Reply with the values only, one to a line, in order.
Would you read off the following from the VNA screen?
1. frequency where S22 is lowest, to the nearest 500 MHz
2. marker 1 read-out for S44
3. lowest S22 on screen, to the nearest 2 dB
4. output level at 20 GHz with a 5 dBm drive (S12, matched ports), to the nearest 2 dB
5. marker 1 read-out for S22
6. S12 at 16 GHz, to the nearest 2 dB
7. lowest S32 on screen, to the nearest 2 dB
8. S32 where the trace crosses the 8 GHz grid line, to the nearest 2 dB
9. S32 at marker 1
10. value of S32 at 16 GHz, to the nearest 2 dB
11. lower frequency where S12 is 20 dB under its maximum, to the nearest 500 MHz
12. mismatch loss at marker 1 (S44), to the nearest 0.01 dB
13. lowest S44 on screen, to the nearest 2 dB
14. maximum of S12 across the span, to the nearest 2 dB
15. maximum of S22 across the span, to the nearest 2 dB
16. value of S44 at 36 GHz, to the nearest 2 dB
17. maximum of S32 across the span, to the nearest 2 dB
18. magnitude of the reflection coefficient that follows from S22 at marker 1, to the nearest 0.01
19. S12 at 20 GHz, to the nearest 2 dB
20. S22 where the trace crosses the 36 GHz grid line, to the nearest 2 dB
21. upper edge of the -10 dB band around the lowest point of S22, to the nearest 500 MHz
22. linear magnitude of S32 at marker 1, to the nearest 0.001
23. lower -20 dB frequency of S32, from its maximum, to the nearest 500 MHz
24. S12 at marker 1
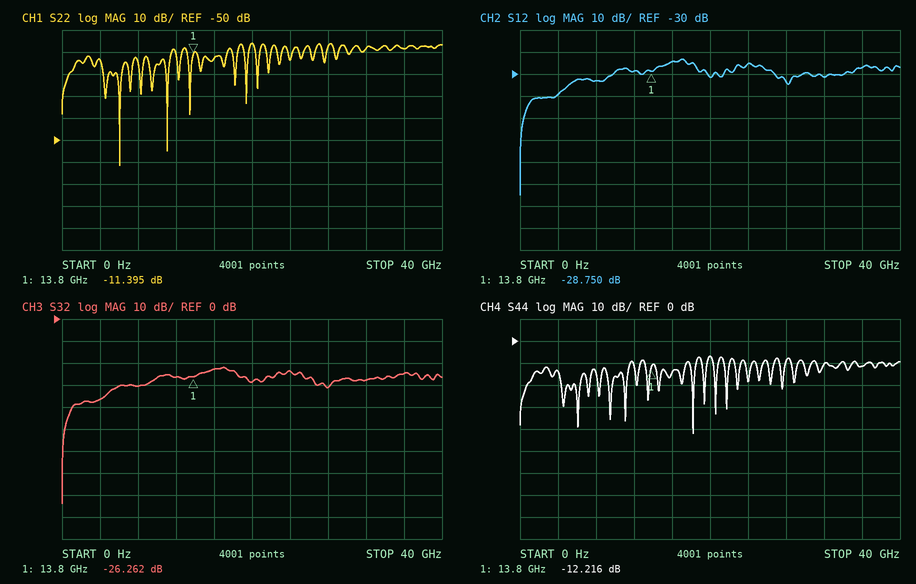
6.0 GHz
-12.216 dB
-62 dB
-26 dBm
-11.395 dB
-24 dB
-84 dB
-30 dB
-26.262 dB
-22 dB
1.0 GHz
0.27 dB
-42 dB
-24 dB
-6 dB
-12 dB
-22 dB
0.27
-32 dB
-8 dB
11.5 GHz
0.049
1.0 GHz
-28.750 dB
